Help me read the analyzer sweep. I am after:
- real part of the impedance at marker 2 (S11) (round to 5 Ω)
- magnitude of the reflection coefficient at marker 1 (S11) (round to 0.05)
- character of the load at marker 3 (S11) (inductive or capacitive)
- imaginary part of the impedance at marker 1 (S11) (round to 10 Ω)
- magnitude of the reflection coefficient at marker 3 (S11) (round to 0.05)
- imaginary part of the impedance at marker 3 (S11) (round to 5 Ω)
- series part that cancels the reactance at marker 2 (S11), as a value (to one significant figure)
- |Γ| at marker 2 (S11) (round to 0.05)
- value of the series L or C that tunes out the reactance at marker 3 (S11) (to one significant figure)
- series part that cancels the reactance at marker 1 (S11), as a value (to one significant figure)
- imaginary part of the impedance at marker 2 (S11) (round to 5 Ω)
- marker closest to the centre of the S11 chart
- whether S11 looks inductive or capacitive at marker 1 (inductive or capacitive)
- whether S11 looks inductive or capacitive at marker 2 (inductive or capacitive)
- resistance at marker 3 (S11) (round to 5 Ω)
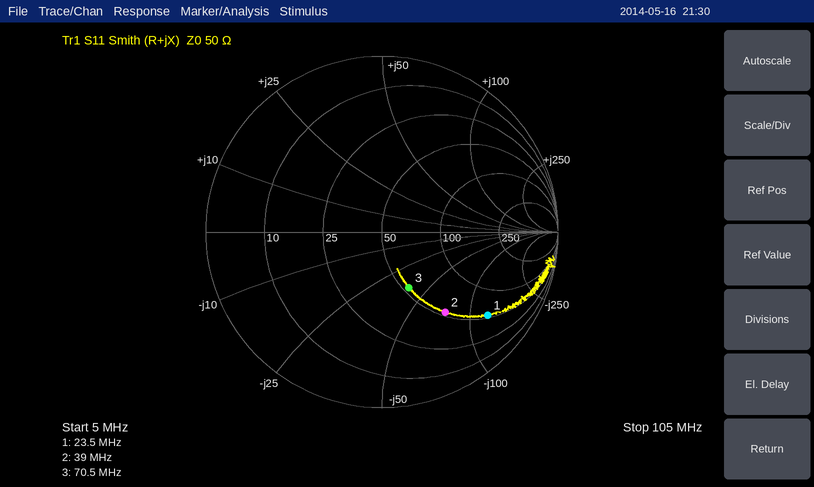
55 Ω
0.75
capacitive
-120 Ω
0.35
-40 Ω
300 nH
0.60
90 nH
800 nH
-75 Ω
marker 3
capacitive
capacitive
55 Ω
